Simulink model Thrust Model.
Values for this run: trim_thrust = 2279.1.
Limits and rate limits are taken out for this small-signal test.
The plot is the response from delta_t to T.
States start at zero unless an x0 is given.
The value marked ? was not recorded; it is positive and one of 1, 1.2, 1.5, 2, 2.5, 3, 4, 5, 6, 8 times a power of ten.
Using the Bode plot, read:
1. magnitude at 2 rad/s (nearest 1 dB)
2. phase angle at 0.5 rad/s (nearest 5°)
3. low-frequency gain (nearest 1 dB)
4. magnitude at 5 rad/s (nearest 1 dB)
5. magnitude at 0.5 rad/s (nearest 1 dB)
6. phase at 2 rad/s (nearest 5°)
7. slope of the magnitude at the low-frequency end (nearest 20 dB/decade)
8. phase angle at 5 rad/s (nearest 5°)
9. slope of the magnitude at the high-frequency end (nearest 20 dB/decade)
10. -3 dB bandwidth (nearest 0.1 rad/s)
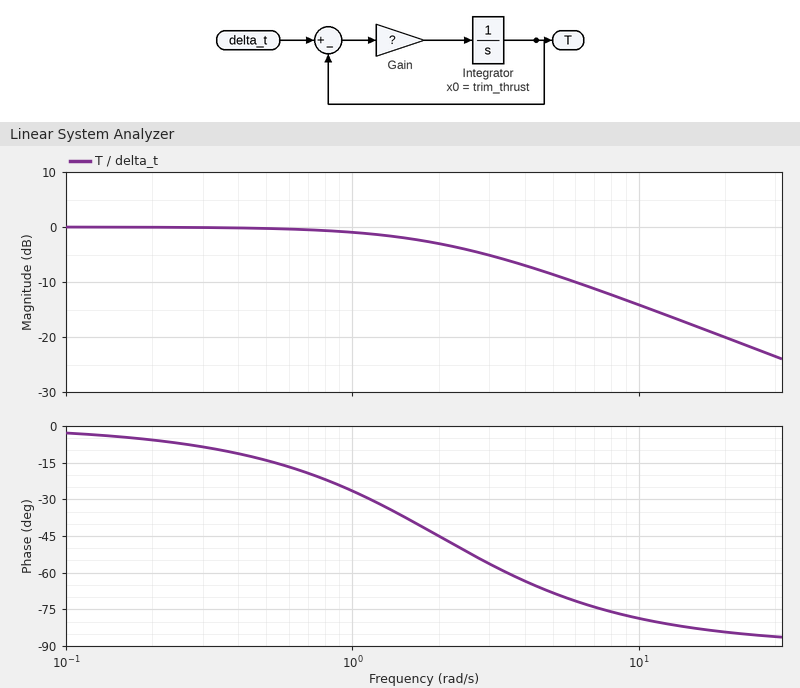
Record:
-3 dB
-15°
0 dB
-9 dB
0 dB
-45°
0 dB/decade
-70°
-20 dB/decade
2.0 rad/s
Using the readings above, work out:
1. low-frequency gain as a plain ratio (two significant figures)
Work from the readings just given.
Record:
1.0
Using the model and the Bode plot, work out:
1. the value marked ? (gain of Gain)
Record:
2
